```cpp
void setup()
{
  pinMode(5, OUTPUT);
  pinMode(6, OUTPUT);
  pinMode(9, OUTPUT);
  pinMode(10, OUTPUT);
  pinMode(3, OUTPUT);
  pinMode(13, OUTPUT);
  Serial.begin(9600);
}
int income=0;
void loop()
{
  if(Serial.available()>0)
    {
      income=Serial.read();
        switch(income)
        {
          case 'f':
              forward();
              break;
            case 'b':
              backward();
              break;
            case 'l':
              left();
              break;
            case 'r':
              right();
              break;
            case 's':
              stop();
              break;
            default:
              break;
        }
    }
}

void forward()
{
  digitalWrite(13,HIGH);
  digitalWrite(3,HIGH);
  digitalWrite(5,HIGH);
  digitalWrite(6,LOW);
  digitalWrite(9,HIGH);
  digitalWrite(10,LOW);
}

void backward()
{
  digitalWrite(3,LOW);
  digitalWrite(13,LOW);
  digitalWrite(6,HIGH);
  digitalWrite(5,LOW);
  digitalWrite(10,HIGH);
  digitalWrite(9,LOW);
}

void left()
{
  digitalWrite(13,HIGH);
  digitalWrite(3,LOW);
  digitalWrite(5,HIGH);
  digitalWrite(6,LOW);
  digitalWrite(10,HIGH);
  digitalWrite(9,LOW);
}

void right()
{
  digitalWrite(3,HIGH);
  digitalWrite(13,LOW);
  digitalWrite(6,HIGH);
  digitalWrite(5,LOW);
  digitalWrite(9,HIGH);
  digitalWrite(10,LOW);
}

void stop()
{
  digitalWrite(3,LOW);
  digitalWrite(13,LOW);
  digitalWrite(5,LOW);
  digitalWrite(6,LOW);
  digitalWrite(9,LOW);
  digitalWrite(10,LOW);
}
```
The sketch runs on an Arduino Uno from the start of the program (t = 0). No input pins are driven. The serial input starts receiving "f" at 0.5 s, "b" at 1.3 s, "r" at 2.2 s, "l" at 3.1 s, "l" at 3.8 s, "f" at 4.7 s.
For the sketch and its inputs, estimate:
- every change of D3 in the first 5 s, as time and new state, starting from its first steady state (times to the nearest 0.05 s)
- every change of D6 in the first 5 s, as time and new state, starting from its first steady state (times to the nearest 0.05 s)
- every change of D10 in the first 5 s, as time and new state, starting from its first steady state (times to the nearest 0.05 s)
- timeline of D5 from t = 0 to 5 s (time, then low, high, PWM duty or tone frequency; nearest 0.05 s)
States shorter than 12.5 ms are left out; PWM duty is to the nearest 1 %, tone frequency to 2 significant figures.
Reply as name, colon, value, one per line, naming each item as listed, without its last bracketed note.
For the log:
every change of D3 in the first 5 s, as time and new state, starting from its first steady state: 0 s low; 0.5 s high; 1.3 s low; 2.2 s high; 3.1 s low; 4.7 s high
every change of D6 in the first 5 s, as time and new state, starting from its first steady state: 0 s low; 1.3 s high; 3.1 s low
every change of D10 in the first 5 s, as time and new state, starting from its first steady state: 0 s low; 1.3 s high; 2.2 s low; 3.1 s high; 4.7 s low
timeline of D5 from t = 0 to 5 s: 0 s low; 0.5 s high; 1.3 s low; 3.1 s high
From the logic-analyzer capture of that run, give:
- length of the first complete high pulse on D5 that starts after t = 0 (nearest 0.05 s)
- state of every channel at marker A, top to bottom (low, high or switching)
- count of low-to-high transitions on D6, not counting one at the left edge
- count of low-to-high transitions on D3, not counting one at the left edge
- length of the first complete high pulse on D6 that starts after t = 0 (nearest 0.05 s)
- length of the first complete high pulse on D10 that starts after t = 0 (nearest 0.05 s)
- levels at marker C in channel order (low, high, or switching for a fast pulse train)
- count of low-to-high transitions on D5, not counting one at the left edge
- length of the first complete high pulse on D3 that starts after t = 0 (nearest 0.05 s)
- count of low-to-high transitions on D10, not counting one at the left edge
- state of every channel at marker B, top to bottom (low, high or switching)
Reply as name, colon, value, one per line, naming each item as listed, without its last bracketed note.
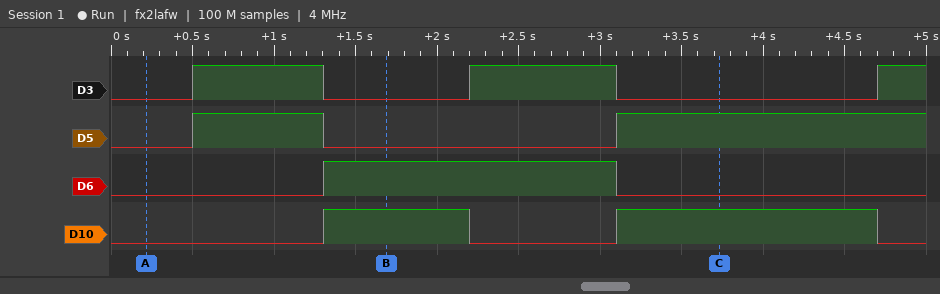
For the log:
length of the first complete high pulse on D5 that starts after t = 0: 0.80 s
state of every channel at marker A, top to bottom: D3 low, D5 low, D6 low, D10 low
count of low-to-high transitions on D6, not counting one at the left edge: 1
count of low-to-high transitions on D3, not counting one at the left edge: 3
length of the first complete high pulse on D6 that starts after t = 0: 1.80 s
length of the first complete high pulse on D10 that starts after t = 0: 0.90 s
levels at marker C in channel order: D3 low, D5 high, D6 low, D10 high
count of low-to-high transitions on D5, not counting one at the left edge: 2
length of the first complete high pulse on D3 that starts after t = 0: 0.80 s
count of low-to-high transitions on D10, not counting one at the left edge: 2
state of every channel at marker B, top to bottom: D3 low, D5 low, D6 high, D10 high
